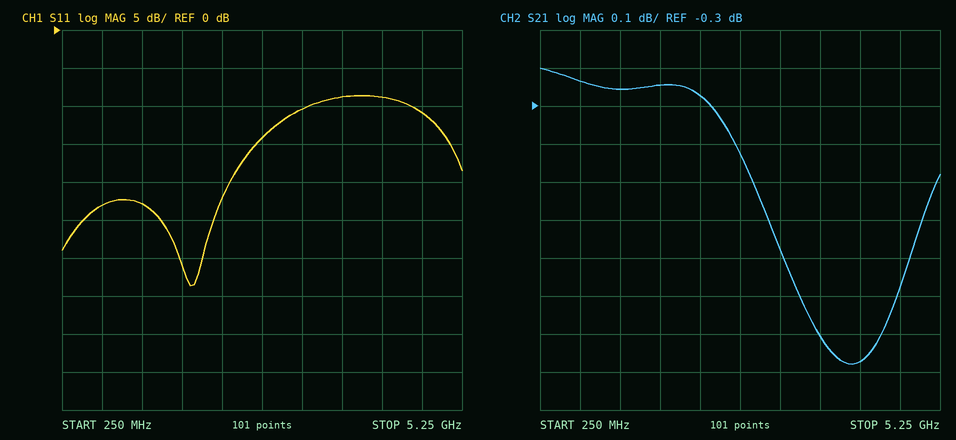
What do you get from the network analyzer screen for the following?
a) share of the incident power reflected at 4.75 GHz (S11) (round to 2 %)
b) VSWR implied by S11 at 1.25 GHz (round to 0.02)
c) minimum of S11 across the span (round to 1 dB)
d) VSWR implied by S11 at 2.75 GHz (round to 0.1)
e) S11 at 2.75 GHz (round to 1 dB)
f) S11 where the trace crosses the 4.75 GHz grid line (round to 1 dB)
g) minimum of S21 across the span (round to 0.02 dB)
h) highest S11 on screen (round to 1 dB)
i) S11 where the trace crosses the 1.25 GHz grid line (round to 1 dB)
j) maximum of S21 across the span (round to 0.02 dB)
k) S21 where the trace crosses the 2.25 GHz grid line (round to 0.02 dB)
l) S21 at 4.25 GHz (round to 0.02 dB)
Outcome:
8 %
1.16
-34 dB
1.5
-14 dB
-11 dB
-0.98 dB
-9 dB
-23 dB
-0.20 dB
-0.28 dB
-0.98 dB
